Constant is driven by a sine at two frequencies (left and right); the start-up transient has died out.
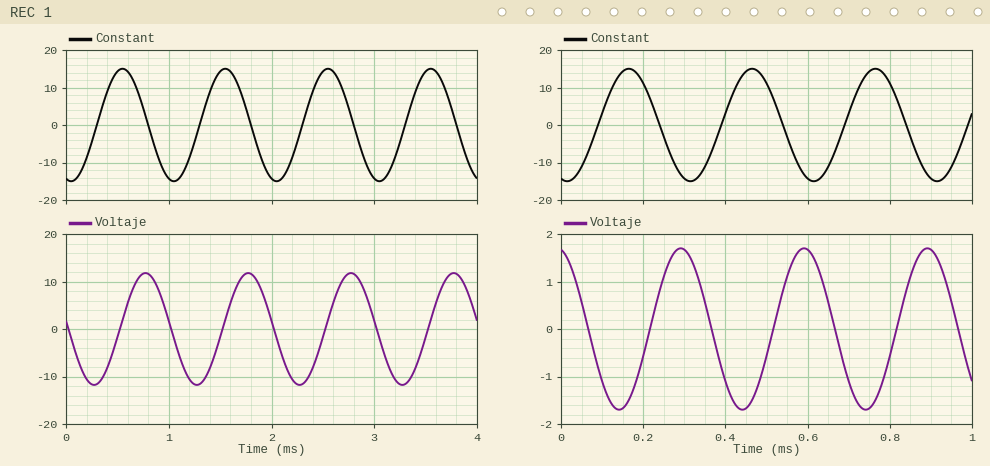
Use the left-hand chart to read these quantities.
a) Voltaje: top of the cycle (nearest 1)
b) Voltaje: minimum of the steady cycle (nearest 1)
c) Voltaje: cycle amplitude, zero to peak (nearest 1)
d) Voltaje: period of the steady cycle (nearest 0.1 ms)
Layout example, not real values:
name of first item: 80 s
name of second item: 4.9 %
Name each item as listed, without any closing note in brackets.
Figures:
Voltaje: top of the cycle: 12
Voltaje: minimum of the steady cycle: -12
Voltaje: cycle amplitude, zero to peak: 12
Voltaje: period of the steady cycle: 1.0 ms
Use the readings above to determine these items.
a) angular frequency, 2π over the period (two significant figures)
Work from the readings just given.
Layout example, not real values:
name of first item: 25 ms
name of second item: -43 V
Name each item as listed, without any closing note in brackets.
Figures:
angular frequency, 2π over the period: 6.3 rad/ms
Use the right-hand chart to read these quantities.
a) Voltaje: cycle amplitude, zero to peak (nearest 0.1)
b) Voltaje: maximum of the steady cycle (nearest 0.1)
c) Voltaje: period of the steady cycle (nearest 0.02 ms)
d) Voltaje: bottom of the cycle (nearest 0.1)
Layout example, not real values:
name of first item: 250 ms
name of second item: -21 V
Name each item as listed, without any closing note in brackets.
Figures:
Voltaje: cycle amplitude, zero to peak: 1.7
Voltaje: maximum of the steady cycle: 1.7
Voltaje: period of the steady cycle: 0.30 ms
Voltaje: bottom of the cycle: -1.7
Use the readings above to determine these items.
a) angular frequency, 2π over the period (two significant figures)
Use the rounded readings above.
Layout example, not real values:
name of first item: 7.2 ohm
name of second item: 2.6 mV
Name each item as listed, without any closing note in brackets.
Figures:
angular frequency, 2π over the period: 21 rad/ms
